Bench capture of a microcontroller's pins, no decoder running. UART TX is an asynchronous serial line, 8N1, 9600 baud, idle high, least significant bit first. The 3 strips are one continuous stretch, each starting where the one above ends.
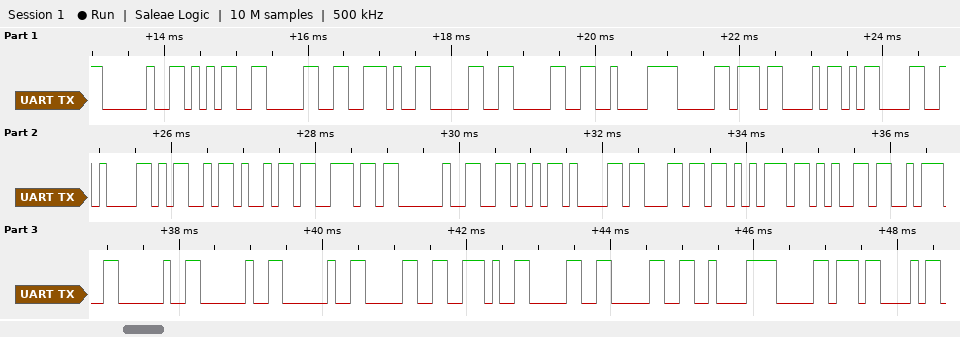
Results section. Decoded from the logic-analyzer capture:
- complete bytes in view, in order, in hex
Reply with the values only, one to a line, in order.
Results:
20 35 30 2E 30 30 C2 B0 43 0D 0A 4D 69 6E 20 56 61 6C 75 65 3A 20 20 20 30 2E 30 30 C2 B0 43
